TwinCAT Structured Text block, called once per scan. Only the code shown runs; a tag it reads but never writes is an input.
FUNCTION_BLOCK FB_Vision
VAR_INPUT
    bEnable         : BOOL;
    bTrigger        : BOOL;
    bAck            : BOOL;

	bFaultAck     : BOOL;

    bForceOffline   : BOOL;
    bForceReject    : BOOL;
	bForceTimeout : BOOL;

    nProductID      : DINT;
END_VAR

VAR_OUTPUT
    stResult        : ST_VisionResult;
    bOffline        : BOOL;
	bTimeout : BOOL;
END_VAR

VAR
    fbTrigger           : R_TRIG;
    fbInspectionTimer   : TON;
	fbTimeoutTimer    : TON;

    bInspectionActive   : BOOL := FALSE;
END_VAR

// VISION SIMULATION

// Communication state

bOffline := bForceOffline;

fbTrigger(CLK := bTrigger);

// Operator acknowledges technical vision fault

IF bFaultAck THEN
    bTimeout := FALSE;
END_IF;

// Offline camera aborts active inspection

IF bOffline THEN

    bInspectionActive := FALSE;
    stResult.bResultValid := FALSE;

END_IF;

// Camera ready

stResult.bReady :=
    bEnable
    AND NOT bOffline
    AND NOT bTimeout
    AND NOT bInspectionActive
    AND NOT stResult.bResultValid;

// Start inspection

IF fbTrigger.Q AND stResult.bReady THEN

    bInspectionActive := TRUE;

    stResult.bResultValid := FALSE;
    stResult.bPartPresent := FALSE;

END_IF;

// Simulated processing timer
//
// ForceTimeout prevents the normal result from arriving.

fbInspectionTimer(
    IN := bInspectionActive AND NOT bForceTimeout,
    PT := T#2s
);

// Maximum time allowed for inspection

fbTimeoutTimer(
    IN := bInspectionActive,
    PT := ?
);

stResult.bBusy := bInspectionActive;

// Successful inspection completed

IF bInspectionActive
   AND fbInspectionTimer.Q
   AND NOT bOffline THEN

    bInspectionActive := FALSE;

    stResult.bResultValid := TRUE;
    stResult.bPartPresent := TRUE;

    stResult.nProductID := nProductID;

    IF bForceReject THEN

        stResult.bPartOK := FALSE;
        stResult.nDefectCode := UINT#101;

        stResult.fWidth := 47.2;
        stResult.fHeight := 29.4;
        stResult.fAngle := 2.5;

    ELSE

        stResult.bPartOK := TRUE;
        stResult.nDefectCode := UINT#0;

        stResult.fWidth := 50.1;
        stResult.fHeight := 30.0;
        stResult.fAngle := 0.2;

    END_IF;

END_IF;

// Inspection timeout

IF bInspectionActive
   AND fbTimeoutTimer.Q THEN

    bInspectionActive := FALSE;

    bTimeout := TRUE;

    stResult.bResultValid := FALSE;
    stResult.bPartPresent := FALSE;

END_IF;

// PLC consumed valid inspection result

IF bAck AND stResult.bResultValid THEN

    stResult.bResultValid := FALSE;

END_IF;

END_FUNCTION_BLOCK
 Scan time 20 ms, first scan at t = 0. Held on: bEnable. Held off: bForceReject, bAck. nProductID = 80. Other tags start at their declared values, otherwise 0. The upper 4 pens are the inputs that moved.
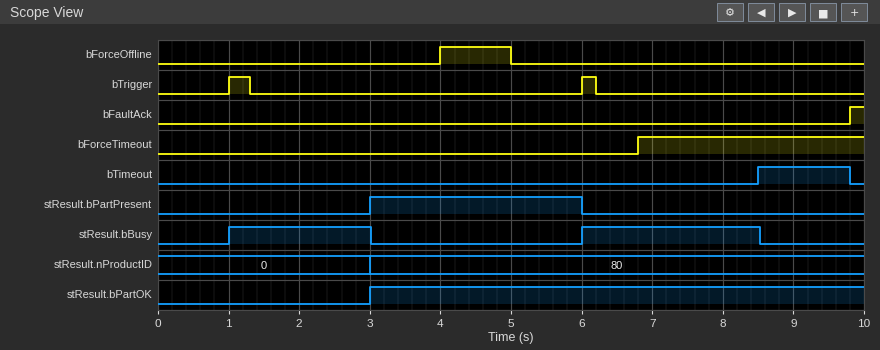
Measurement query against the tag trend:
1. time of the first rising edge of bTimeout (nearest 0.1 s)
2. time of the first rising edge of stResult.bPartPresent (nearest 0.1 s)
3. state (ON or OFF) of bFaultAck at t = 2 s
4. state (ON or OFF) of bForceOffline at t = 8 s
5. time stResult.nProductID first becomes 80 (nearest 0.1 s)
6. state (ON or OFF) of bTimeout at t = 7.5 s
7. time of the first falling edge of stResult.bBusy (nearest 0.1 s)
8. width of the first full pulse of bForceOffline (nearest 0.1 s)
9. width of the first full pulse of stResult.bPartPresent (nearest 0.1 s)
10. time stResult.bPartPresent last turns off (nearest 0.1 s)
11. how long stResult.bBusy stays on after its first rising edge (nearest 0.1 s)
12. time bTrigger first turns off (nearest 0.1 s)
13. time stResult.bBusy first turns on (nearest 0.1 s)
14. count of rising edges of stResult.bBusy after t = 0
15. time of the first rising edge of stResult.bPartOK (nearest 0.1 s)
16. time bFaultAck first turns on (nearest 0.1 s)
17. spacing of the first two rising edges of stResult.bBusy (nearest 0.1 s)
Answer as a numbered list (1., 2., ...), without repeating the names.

1. 8.5 s
2. 3.0 s
3. OFF
4. OFF
5. 3.0 s
6. OFF
7. 3.0 s
8. 1.0 s
9. 3.0 s
10. 6.0 s
11. 2.0 s
12. 1.3 s
13. 1.0 s
14. 2
15. 3.0 s
16. 9.8 s
17. 5.0 s
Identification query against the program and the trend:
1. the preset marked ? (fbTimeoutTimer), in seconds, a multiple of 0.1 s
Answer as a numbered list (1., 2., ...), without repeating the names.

1. 2.5 s
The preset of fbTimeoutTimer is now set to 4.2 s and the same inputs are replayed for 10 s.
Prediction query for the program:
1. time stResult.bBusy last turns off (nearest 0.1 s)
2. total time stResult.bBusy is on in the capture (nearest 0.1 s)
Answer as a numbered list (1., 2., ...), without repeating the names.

1. 3.0 s
2. 6.0 s
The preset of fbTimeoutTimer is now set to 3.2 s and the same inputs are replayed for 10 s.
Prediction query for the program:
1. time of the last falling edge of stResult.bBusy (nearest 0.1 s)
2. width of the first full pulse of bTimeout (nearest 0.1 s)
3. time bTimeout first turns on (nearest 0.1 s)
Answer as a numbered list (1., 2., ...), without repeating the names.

1. 9.2 s
2. 0.6 s
3. 9.2 s
